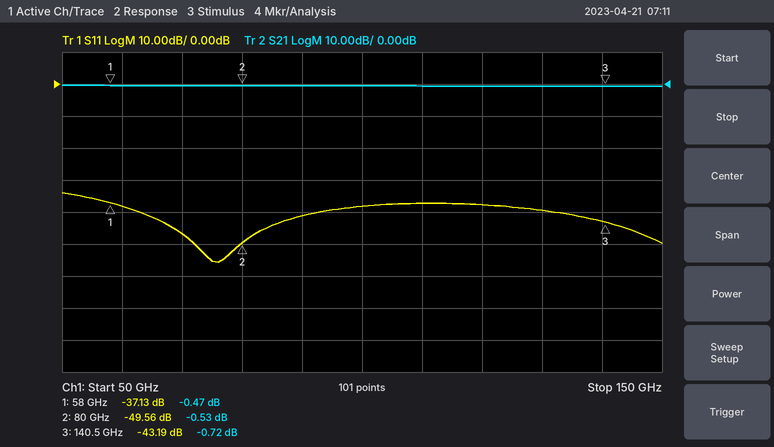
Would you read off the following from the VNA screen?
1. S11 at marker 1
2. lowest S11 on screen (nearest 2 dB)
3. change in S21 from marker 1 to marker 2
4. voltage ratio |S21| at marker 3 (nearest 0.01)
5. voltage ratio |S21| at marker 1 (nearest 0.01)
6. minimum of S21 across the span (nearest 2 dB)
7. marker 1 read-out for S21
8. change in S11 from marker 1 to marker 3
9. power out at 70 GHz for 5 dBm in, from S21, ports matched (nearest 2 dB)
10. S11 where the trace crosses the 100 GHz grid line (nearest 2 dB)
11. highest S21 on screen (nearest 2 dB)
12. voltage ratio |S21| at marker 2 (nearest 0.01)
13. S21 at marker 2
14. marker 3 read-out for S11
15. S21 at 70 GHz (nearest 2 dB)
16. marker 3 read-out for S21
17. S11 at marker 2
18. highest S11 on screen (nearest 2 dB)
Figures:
-37.13 dB
-56 dB
-0.06 dB
0.92
0.95
0 dB
-0.47 dB
-6.06 dB
4 dBm
-38 dB
0 dB
0.94
-0.53 dB
-43.19 dB
0 dB
-0.72 dB
-49.56 dB
-34 dB
